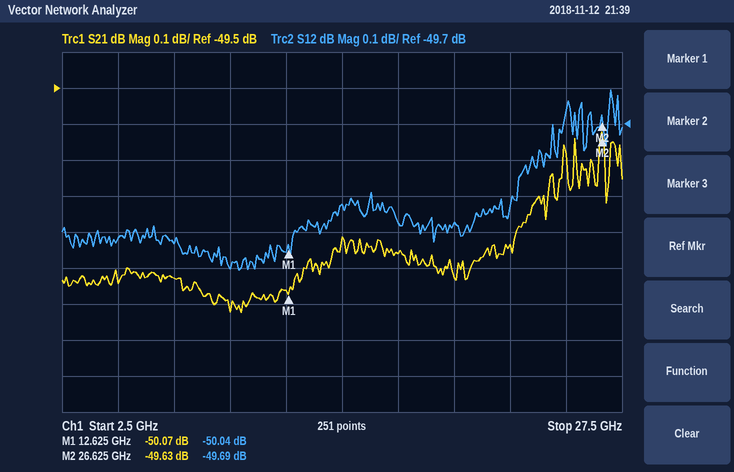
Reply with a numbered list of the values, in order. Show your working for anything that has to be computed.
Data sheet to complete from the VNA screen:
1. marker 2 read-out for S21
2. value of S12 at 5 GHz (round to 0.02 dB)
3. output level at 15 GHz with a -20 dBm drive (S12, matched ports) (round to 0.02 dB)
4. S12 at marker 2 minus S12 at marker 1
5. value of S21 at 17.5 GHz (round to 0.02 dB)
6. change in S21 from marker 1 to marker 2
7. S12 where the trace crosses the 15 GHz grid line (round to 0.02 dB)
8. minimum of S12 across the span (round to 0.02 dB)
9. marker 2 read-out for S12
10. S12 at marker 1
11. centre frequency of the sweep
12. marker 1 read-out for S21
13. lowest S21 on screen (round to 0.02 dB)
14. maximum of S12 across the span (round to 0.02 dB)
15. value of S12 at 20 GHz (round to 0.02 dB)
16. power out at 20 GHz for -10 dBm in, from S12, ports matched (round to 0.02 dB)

1. -49.63 dB
2. -50.02 dB
3. -20 dBm + (-49.92 dB) = -69.92 dBm
4. -49.69 − (-50.04) = 0.35 dB
5. -49.96 dB
6. -49.63 − (-50.07) = 0.44 dB
7. -49.92 dB
8. -50.10 dB
9. -49.69 dB
10. -50.04 dB
11. 15 GHz
12. -50.07 dB
13. -50.12 dB
14. -49.60 dB
15. -49.98 dB
16. -10 dBm + (-49.98 dB) = -59.98 dBm
